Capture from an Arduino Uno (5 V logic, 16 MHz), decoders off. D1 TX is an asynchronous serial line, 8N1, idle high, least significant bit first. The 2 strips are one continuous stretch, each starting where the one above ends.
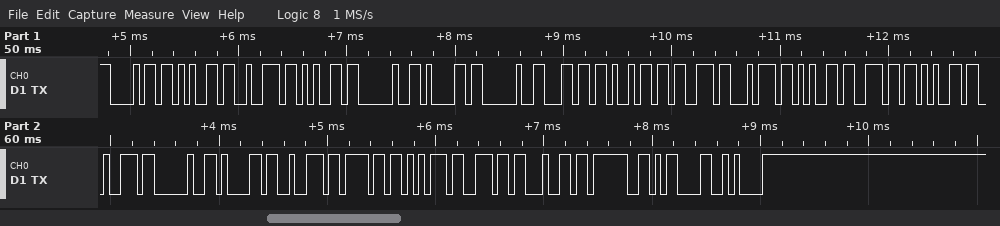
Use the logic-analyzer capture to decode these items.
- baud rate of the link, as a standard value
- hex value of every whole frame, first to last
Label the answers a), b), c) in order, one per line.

a) 19200 baud
b) 68 65 72 65 20 61 20 6C 69 73 74 65 6E 65 72 20 61 72 6F 75 6E 64 3F 0D 0A
